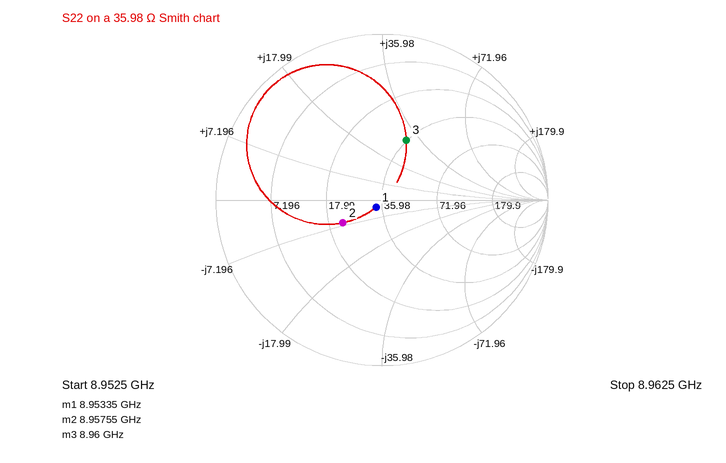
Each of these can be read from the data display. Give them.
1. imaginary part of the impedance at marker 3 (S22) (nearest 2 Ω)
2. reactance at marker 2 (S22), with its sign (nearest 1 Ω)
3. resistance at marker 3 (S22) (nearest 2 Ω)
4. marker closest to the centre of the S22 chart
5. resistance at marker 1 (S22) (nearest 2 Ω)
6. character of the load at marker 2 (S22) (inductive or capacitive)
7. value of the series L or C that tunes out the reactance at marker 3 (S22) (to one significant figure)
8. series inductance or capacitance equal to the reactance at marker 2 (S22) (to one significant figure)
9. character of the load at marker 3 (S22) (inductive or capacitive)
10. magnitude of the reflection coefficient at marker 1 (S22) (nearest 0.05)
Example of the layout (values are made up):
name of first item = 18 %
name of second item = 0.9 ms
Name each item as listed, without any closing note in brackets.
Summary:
imaginary part of the impedance at marker 3 (S22) = +30 Ω
reactance at marker 2 (S22), with its sign = -6 Ω
resistance at marker 3 (S22) = 36 Ω
marker closest to the centre of the S22 chart = marker 1
resistance at marker 1 (S22) = 34 Ω
character of the load at marker 2 (S22) = capacitive
value of the series L or C that tunes out the reactance at marker 3 (S22) = 600 fF
series inductance or capacitance equal to the reactance at marker 2 (S22) = 3 pF
character of the load at marker 3 (S22) = inductive
magnitude of the reflection coefficient at marker 1 (S22) = 0.05
